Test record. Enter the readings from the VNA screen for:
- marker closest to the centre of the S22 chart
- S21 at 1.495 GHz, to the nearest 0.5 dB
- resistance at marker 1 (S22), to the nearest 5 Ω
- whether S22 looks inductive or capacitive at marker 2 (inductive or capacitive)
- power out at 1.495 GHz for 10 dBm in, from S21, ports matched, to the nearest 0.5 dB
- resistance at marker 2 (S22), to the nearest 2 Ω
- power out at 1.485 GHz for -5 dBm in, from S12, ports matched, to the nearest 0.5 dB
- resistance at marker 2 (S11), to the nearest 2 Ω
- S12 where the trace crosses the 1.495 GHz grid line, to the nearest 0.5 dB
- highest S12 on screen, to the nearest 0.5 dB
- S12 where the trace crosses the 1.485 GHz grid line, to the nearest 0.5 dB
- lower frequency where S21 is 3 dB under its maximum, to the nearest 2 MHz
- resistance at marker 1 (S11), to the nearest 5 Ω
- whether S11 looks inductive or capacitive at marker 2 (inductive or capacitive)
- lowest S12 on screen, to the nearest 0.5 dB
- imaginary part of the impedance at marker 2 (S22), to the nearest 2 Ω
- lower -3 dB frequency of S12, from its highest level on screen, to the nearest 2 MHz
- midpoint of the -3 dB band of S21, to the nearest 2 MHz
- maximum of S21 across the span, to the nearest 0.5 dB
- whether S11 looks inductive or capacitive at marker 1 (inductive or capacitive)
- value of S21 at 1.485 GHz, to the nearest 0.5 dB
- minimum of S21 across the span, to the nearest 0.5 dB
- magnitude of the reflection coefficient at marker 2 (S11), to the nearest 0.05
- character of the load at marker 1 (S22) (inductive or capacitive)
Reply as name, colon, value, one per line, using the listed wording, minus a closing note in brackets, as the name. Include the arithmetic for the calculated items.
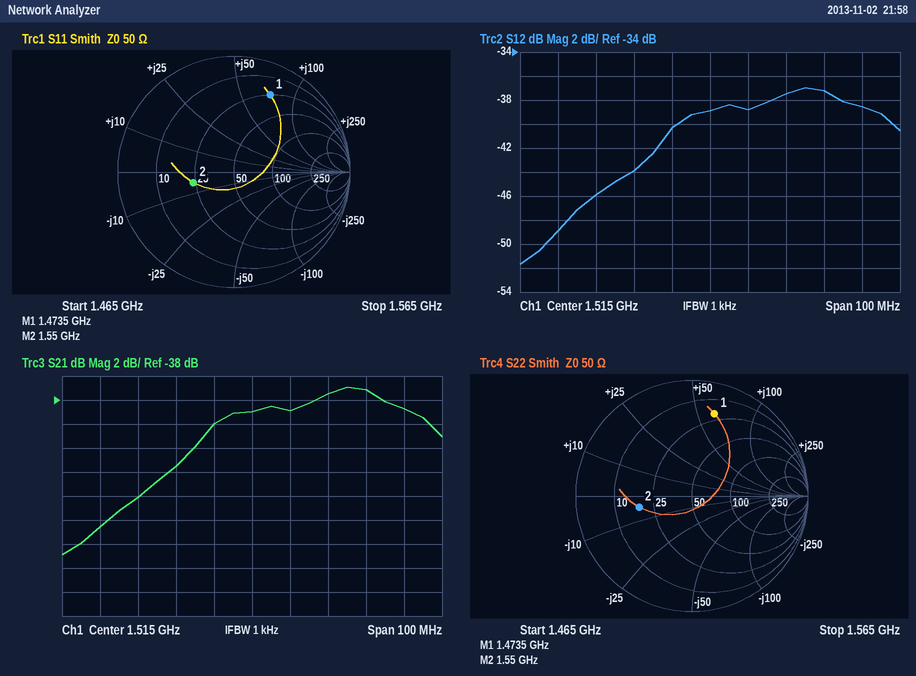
marker closest to the centre of the S22 chart: marker 2
S21 at 1.495 GHz, to the nearest 0.5 dB: -43.5 dB
resistance at marker 1 (S22), to the nearest 5 Ω: 20 Ω
whether S22 looks inductive or capacitive at marker 2: capacitive
power out at 1.495 GHz for 10 dBm in, from S21, ports matched, to the nearest 0.5 dB: 10 dBm + (-43.5 dB) = -33.5 dBm
resistance at marker 2 (S22), to the nearest 2 Ω: 18 Ω
power out at 1.485 GHz for -5 dBm in, from S12, ports matched, to the nearest 0.5 dB: -5 dBm + (-46.0 dB) = -51.0 dBm
resistance at marker 2 (S11), to the nearest 2 Ω: 24 Ω
S12 where the trace crosses the 1.495 GHz grid line, to the nearest 0.5 dB: -44.0 dB
highest S12 on screen, to the nearest 0.5 dB: -37.0 dB
S12 where the trace crosses the 1.485 GHz grid line, to the nearest 0.5 dB: -46.0 dB
lower frequency where S21 is 3 dB under its maximum, to the nearest 2 MHz: 1.506 GHz
resistance at marker 1 (S11), to the nearest 5 Ω: 25 Ω
whether S11 looks inductive or capacitive at marker 2: capacitive
lowest S12 on screen, to the nearest 0.5 dB: -51.5 dB
imaginary part of the impedance at marker 2 (S22), to the nearest 2 Ω: -4 Ω
lower -3 dB frequency of S12, from its highest level on screen, to the nearest 2 MHz: 1.506 GHz
midpoint of the -3 dB band of S21, to the nearest 2 MHz: 1.534 GHz
maximum of S21 across the span, to the nearest 0.5 dB: -37.0 dB
whether S11 looks inductive or capacitive at marker 1: inductive
value of S21 at 1.485 GHz, to the nearest 0.5 dB: -46.0 dB
minimum of S21 across the span, to the nearest 0.5 dB: -51.0 dB
magnitude of the reflection coefficient at marker 2 (S11), to the nearest 0.05: 0.35
character of the load at marker 1 (S22): inductive
